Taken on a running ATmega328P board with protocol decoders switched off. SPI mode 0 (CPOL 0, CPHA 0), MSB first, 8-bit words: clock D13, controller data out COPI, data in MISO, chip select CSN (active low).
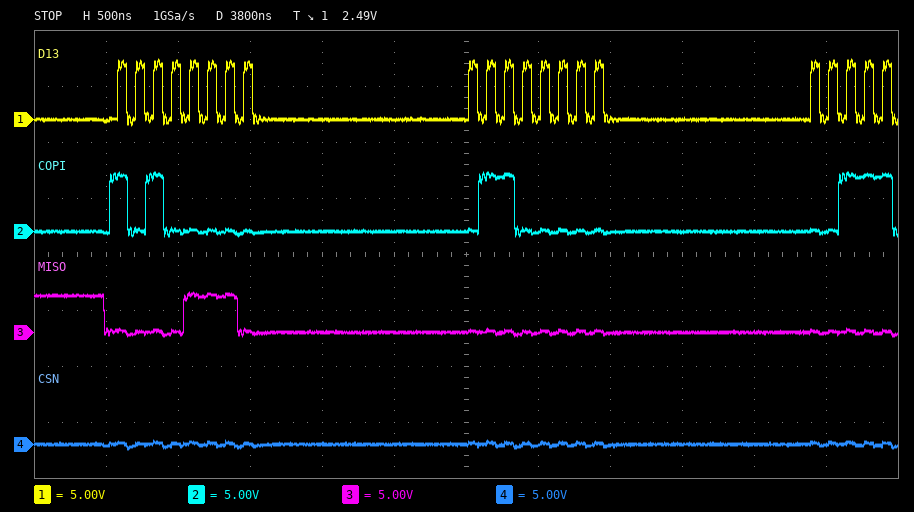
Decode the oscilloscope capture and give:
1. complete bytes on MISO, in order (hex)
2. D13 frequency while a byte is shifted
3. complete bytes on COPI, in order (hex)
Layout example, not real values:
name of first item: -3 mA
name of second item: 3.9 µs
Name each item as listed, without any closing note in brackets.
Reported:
complete bytes on MISO, in order: 0E 00
D13 frequency while a byte is shifted: 8 MHz
complete bytes on COPI, in order: A0 60
